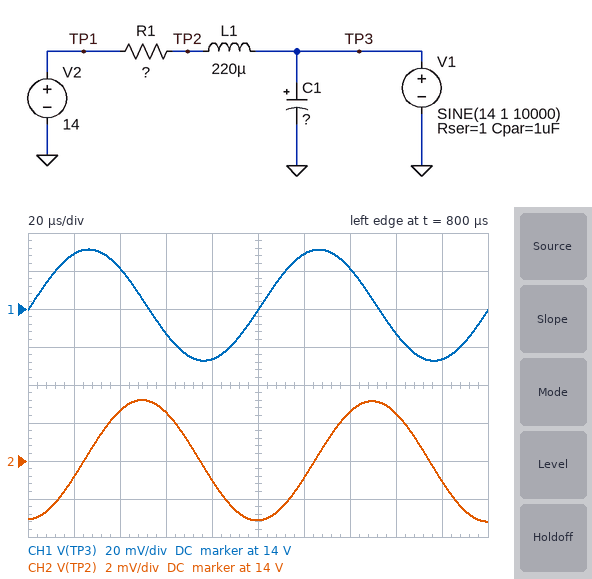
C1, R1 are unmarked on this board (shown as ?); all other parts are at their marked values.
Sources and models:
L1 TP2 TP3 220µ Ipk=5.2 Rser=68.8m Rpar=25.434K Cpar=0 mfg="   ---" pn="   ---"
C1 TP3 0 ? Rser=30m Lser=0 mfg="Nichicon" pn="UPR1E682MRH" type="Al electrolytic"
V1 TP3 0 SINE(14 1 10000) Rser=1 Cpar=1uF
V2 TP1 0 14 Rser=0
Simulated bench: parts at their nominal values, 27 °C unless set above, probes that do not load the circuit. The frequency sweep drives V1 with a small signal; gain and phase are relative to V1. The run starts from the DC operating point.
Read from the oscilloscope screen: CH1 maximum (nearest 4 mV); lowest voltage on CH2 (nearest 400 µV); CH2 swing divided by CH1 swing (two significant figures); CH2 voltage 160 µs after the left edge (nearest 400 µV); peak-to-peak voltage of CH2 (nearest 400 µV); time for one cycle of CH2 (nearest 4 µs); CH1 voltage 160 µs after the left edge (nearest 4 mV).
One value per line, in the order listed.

14.032 V
13.9988 V
0.11
14.0044 V
6.4 mV
100 µs
13.988 V
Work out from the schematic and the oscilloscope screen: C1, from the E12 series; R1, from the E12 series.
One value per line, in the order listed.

5.6 mF
1.5 Ω
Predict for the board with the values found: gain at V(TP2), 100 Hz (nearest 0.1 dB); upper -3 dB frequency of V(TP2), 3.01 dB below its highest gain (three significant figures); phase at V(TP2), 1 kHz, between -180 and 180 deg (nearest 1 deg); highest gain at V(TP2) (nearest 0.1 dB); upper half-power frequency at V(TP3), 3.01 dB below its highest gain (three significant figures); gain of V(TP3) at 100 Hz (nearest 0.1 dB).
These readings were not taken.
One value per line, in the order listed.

-12.4 dB
45.1 Hz
-82 deg
-4.7 dB
45.1 Hz
-12.0 dB
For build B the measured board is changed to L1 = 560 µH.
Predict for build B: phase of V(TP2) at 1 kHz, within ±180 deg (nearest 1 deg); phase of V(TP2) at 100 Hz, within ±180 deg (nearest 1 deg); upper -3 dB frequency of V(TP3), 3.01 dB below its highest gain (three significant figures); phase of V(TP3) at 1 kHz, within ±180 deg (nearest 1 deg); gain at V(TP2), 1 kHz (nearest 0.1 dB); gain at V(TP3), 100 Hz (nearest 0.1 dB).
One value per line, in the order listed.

-107 deg
-72 deg
46.3 Hz
-41 deg
-36.1 dB
-11.8 dB
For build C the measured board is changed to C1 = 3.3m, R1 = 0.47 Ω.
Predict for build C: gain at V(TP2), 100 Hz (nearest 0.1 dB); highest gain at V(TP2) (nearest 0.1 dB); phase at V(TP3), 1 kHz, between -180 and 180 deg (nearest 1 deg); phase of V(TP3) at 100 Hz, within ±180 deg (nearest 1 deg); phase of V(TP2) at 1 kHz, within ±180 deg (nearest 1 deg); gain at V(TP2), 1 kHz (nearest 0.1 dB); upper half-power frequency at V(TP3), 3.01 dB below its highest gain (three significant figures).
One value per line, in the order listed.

-11.8 dB
-10.3 dB
-54 deg
-29 deg
-122 deg
-35.0 dB
169 Hz
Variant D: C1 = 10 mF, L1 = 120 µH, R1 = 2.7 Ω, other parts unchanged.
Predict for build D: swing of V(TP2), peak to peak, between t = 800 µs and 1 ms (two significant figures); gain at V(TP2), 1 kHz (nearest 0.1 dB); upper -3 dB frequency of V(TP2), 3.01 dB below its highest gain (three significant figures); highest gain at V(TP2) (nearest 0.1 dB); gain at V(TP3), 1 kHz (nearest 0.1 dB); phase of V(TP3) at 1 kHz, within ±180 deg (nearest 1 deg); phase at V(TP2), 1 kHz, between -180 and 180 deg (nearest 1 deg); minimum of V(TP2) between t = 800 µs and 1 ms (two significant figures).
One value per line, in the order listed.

20 mV
-30.2 dB
20.9 Hz
-2.9 dB
-29.7 dB
-27 deg
-42 deg
14 V
